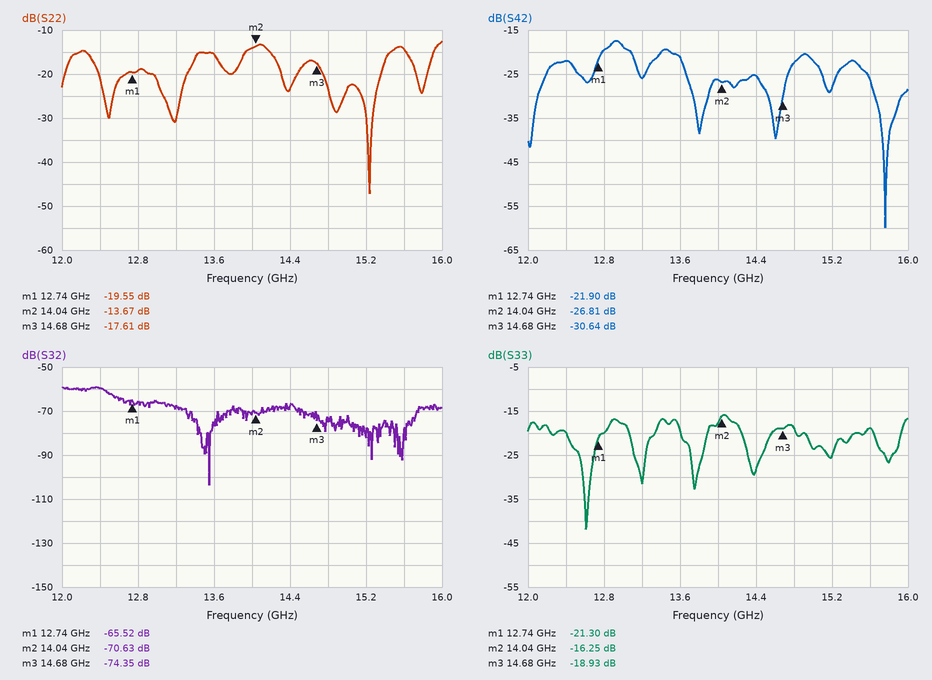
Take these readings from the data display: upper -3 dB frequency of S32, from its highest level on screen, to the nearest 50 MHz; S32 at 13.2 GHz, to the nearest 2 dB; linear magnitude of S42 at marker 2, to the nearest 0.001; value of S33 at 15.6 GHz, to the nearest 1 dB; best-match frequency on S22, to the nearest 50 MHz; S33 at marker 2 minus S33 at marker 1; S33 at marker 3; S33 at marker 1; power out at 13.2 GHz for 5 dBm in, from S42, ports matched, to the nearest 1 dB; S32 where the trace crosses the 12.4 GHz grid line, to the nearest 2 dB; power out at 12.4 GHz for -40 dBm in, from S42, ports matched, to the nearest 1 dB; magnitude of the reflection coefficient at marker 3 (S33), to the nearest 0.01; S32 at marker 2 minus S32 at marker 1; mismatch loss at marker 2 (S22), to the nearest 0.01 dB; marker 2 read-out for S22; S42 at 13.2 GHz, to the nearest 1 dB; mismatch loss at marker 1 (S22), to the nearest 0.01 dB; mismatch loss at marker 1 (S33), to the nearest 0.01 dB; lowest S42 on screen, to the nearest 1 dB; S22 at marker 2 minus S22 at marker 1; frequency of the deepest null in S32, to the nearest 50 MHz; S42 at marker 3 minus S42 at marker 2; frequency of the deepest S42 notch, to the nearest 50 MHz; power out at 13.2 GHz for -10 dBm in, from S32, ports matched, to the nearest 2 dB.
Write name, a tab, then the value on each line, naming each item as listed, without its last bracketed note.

upper -3 dB frequency of S32, from its highest level on screen, to the nearest 50 MHz	12.50 GHz
S32 at 13.2 GHz, to the nearest 2 dB	-68 dB
linear magnitude of S42 at marker 2, to the nearest 0.001	0.046
value of S33 at 15.6 GHz, to the nearest 1 dB	-19 dB
best-match frequency on S22, to the nearest 50 MHz	15.25 GHz
S33 at marker 2 minus S33 at marker 1	5.05 dB
S33 at marker 3	-18.93 dB
S33 at marker 1	-21.30 dB
power out at 13.2 GHz for 5 dBm in, from S42, ports matched, to the nearest 1 dB	-21 dBm
S32 where the trace crosses the 12.4 GHz grid line, to the nearest 2 dB	-60 dB
power out at 12.4 GHz for -40 dBm in, from S42, ports matched, to the nearest 1 dB	-62 dBm
magnitude of the reflection coefficient at marker 3 (S33), to the nearest 0.01	0.11
S32 at marker 2 minus S32 at marker 1	-5.11 dB
mismatch loss at marker 2 (S22), to the nearest 0.01 dB	0.19 dB
marker 2 read-out for S22	-13.67 dB
S42 at 13.2 GHz, to the nearest 1 dB	-26 dB
mismatch loss at marker 1 (S22), to the nearest 0.01 dB	0.05 dB
mismatch loss at marker 1 (S33), to the nearest 0.01 dB	0.03 dB
lowest S42 on screen, to the nearest 1 dB	-60 dB
S22 at marker 2 minus S22 at marker 1	5.88 dB
frequency of the deepest null in S32, to the nearest 50 MHz	13.55 GHz
S42 at marker 3 minus S42 at marker 2	-3.83 dB
frequency of the deepest S42 notch, to the nearest 50 MHz	15.75 GHz
power out at 13.2 GHz for -10 dBm in, from S32, ports matched, to the nearest 2 dB	-78 dBm
